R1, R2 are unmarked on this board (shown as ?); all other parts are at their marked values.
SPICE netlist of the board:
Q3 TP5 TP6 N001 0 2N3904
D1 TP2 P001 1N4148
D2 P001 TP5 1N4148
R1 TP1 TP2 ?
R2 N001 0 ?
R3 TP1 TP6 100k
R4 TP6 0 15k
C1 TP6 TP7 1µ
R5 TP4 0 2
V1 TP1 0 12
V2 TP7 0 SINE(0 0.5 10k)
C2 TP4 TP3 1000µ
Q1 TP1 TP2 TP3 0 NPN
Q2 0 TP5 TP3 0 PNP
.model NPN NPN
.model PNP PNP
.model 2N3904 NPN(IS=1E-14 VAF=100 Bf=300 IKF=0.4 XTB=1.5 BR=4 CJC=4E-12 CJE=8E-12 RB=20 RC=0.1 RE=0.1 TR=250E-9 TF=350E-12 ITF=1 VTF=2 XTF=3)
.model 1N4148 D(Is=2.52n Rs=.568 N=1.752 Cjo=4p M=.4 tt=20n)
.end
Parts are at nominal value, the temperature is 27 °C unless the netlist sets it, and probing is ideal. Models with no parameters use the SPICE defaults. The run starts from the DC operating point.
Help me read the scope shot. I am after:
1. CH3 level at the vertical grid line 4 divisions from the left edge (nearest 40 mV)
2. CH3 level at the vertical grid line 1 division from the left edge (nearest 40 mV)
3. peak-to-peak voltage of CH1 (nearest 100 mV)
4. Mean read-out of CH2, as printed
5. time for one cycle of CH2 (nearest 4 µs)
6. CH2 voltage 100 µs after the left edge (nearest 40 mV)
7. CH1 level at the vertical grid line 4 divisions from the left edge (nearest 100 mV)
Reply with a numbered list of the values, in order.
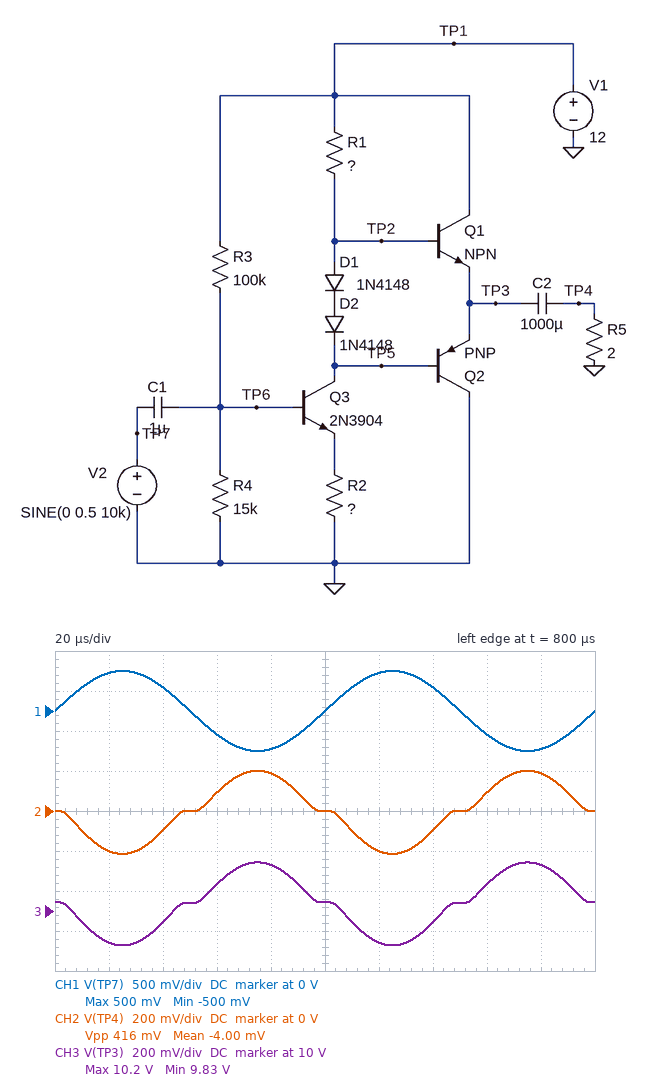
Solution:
1. 10.24 V
2. 9.84 V
3. 1.0 V
4. -4.00 mV
5. 100 µs
6. 0 V
7. -500 mV
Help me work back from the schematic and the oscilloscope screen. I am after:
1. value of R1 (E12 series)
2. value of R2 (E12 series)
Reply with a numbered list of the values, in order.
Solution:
1. 390 Ω
2. 220 Ω
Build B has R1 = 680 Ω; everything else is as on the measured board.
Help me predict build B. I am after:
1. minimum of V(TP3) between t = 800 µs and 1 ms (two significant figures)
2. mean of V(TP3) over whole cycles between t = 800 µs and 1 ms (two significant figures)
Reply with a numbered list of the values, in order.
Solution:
1. 8.8 V
2. 9.1 V
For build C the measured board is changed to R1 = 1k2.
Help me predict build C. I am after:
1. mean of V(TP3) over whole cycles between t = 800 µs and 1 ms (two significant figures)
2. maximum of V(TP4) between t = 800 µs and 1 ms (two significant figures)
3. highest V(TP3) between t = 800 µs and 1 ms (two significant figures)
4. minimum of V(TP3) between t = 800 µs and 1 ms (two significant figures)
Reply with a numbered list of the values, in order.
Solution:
1. 7.3 V
2. 330 mV
3. 7.7 V
4. 7.0 V
